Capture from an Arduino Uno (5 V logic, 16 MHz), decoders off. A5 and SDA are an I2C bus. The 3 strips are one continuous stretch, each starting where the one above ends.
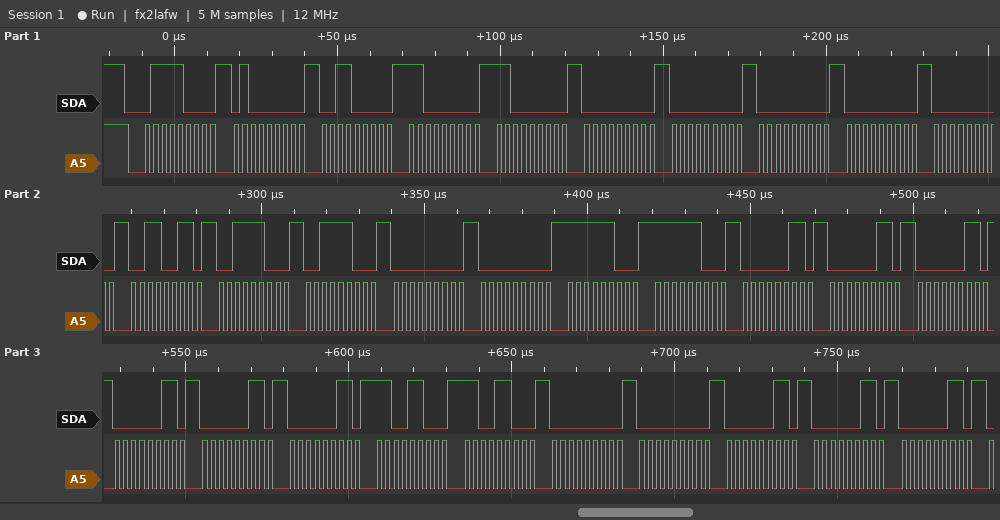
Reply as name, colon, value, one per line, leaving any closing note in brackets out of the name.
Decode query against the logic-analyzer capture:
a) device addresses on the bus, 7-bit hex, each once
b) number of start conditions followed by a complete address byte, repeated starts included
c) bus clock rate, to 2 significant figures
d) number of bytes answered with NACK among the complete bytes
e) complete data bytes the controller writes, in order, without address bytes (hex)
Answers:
device addresses on the bus, 7-bit hex, each once: 0x3C
number of start conditions followed by a complete address byte, repeated starts included: 1
bus clock rate, to 2 significant figures: 400 kHz
number of bytes answered with NACK among the complete bytes: 0
complete data bytes the controller writes, in order, without address bytes: 40 30 C0 C0 00 00 00 00 00 33 3C 3C 00 00 FC FC 03 03 03 03 03 03 CC CC 00 00 03 03 03
